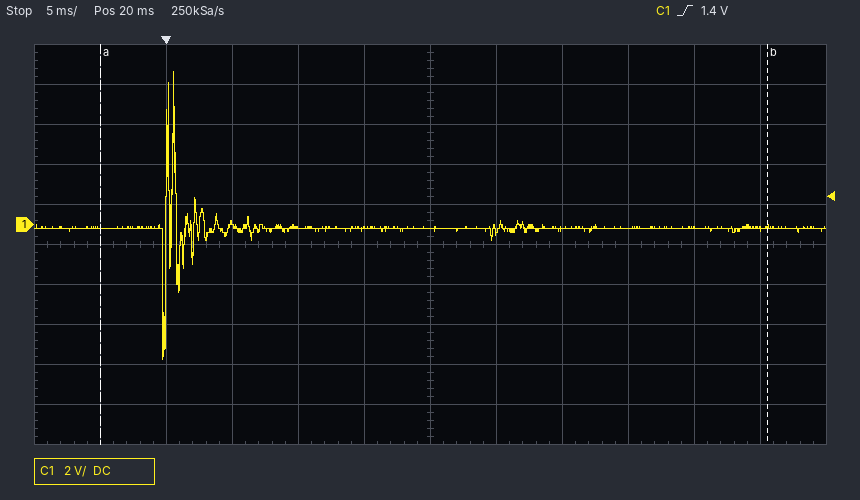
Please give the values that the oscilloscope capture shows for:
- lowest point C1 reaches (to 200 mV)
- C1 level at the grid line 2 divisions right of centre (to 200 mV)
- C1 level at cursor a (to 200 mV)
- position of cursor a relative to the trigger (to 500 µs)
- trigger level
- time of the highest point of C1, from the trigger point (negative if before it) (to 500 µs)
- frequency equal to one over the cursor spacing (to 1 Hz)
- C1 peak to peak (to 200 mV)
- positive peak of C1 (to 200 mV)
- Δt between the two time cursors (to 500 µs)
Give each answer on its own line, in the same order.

-6.8 V
-200 mV
-200 mV
-5.0 ms
1.4 V
+500 µs
20 Hz
14.4 V
7.6 V
50.5 ms
